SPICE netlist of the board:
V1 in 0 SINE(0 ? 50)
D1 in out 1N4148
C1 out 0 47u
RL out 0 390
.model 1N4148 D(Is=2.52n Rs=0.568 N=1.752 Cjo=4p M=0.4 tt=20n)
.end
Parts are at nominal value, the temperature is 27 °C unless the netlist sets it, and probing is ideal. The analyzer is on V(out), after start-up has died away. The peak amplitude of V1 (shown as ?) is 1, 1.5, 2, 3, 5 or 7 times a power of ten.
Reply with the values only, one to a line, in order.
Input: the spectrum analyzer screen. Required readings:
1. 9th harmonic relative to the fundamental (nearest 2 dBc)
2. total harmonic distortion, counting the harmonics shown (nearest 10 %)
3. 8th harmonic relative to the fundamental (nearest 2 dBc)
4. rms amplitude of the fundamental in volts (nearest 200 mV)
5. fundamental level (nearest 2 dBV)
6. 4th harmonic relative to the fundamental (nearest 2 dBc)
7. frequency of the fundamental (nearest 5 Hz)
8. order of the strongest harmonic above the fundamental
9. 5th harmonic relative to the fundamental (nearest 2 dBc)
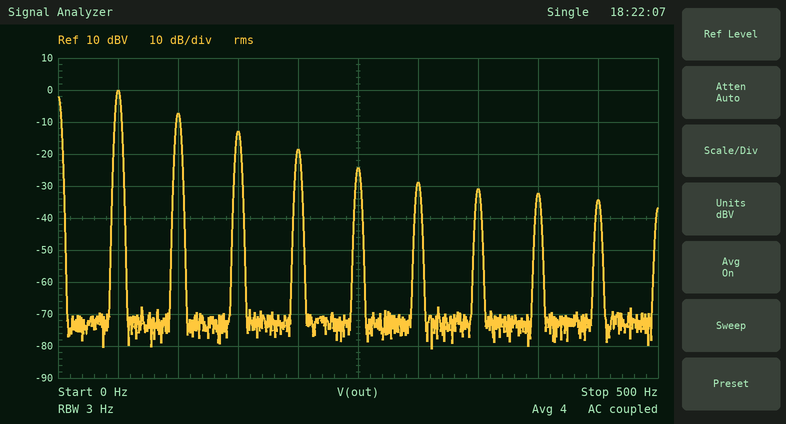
-34 dBc
50 %
-32 dBc
1.0 V
0 dBV
-18 dBc
50 Hz
2
-24 dBc
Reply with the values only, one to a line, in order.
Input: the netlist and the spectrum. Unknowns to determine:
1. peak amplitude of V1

7 V
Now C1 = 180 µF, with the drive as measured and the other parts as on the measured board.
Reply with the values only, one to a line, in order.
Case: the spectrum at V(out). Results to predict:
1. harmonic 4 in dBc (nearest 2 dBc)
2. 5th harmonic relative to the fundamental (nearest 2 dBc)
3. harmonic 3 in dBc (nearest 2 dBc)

-14 dBc
-18 dBc
-10 dBc
